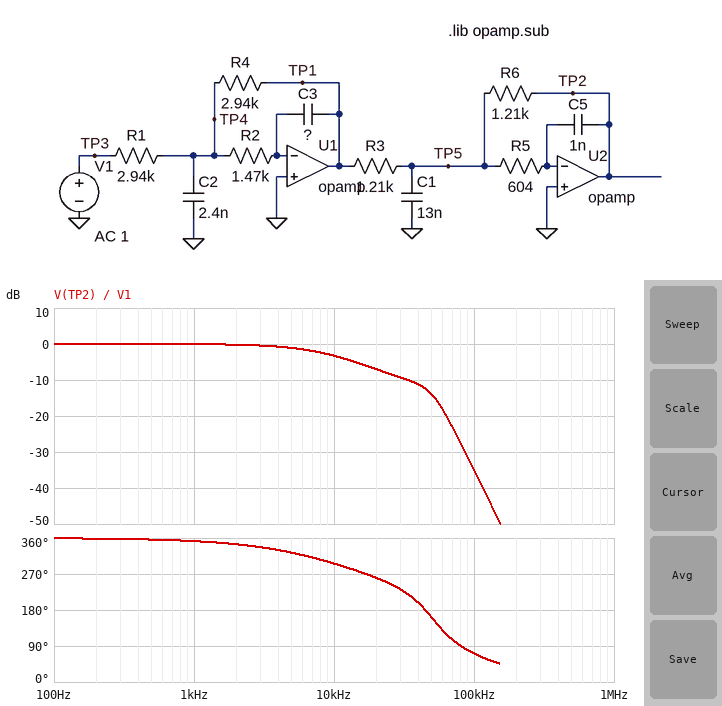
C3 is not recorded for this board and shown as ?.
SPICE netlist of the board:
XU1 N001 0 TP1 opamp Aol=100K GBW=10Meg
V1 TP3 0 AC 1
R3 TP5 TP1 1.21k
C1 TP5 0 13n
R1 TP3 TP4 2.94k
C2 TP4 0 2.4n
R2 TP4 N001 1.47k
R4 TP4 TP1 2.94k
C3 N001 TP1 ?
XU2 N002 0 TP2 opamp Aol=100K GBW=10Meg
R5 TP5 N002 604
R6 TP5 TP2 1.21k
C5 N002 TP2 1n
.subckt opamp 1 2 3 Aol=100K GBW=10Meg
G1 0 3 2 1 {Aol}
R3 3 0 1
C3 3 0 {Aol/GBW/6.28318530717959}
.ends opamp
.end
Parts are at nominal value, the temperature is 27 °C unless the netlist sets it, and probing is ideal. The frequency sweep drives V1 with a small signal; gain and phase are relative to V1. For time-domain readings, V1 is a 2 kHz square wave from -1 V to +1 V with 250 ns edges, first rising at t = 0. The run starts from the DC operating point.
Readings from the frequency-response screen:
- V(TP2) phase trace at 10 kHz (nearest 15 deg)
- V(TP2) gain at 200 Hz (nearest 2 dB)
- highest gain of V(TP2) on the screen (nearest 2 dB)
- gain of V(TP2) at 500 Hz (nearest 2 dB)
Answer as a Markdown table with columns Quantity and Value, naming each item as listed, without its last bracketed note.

| Quantity | Value |
|---|---|
| V(TP2) phase trace at 10 kHz | 300 deg |
| V(TP2) gain at 200 Hz | 0 dB |
| highest gain of V(TP2) on the screen | 0 dB |
| gain of V(TP2) at 500 Hz | 0 dB |
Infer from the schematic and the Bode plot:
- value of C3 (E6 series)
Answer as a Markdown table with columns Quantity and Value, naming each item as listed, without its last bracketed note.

| Quantity | Value |
|---|---|
| value of C3 | 3.3 nF |
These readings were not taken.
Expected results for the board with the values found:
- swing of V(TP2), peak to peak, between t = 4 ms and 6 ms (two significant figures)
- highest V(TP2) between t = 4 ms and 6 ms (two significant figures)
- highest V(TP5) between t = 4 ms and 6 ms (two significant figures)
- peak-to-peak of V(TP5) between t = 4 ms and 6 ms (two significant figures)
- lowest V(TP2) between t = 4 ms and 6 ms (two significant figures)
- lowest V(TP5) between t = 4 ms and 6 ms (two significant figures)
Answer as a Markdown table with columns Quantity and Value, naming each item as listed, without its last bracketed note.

| Quantity | Value |
|---|---|
| swing of V(TP2), peak to peak, between t = 4 ms and 6 ms | 2.0 V |
| highest V(TP2) between t = 4 ms and 6 ms | 1.0 V |
| highest V(TP5) between t = 4 ms and 6 ms | 63 mV |
| peak-to-peak of V(TP5) between t = 4 ms and 6 ms | 130 mV |
| lowest V(TP2) between t = 4 ms and 6 ms | -1.0 V |
| lowest V(TP5) between t = 4 ms and 6 ms | -63 mV |
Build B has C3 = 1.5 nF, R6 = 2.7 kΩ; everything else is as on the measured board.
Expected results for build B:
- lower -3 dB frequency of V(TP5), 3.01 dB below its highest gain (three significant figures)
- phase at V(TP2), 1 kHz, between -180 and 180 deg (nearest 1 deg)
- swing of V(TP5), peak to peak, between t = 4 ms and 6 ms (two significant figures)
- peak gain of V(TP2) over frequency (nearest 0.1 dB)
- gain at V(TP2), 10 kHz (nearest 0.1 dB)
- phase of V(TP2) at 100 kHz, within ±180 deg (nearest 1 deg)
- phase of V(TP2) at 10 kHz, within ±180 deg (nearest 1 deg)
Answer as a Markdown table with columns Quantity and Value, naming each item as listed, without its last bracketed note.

| Quantity | Value |
|---|---|
| lower -3 dB frequency of V(TP5), 3.01 dB below its highest gain | 15.0 kHz |
| phase at V(TP2), 1 kHz, between -180 and 180 deg | -5 deg |
| swing of V(TP5), peak to peak, between t = 4 ms and 6 ms | 390 mV |
| peak gain of V(TP2) over frequency | 7.0 dB |
| gain at V(TP2), 10 kHz | 6.6 dB |
| phase of V(TP2) at 100 kHz, within ±180 deg | 67 deg |
| phase of V(TP2) at 10 kHz, within ±180 deg | -49 deg |
